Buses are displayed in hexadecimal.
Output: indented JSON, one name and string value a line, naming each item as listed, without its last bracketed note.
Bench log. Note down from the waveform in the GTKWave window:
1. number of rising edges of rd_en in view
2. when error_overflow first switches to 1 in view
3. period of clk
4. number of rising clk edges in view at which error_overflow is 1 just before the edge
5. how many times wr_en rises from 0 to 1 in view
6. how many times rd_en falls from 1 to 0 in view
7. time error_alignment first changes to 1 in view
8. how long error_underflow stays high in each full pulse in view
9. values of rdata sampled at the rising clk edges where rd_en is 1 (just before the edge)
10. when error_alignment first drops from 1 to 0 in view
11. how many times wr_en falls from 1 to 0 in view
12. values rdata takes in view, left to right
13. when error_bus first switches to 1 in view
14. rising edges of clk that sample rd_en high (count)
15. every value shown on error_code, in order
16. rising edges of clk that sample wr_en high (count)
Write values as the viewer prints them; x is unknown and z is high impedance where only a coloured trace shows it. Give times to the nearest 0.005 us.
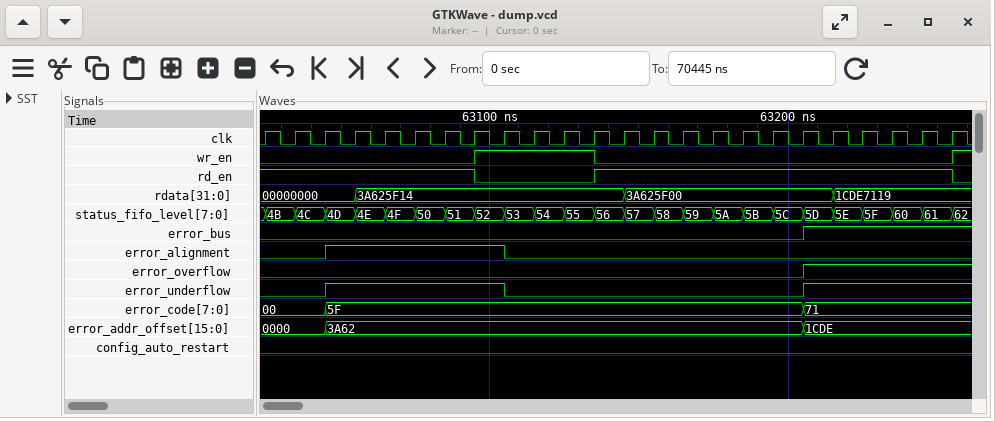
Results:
{
  "number of rising edges of rd_en in view": "1",
  "when error_overflow first switches to 1 in view": "63.205 us",
  "period of clk": "0.01 us",
  "number of rising clk edges in view at which error_overflow is 1 just before the edge": "5",
  "how many times wr_en rises from 0 to 1 in view": "2",
  "how many times rd_en falls from 1 to 0 in view": "2",
  "time error_alignment first changes to 1 in view": "63.045 us",
  "how long error_underflow stays high in each full pulse in view": "0.06 us",
  "values of rdata sampled at the rising clk edges where rd_en is 1": "00000000, 00000000, 00000000, 00000000, 3A625F14, 3A625F14, 3A625F14, 3A625F14, 3A625F14, 3A625F00, 3A625F00, 3A625F00, 3A625F00, 3A625F00, 3A625F00, 3A625F00, 1CDE7119, 1CDE7119, 1CDE7119, 1CDE7119",
  "when error_alignment first drops from 1 to 0 in view": "63.105 us",
  "how many times wr_en falls from 1 to 0 in view": "1",
  "values rdata takes in view, left to right": "00000000, 3A625F14, 3A625F00, 1CDE7119",
  "when error_bus first switches to 1 in view": "63.205 us",
  "rising edges of clk that sample rd_en high": "20",
  "every value shown on error_code, in order": "00, 5F, 71",
  "rising edges of clk that sample wr_en high": "4"
}
